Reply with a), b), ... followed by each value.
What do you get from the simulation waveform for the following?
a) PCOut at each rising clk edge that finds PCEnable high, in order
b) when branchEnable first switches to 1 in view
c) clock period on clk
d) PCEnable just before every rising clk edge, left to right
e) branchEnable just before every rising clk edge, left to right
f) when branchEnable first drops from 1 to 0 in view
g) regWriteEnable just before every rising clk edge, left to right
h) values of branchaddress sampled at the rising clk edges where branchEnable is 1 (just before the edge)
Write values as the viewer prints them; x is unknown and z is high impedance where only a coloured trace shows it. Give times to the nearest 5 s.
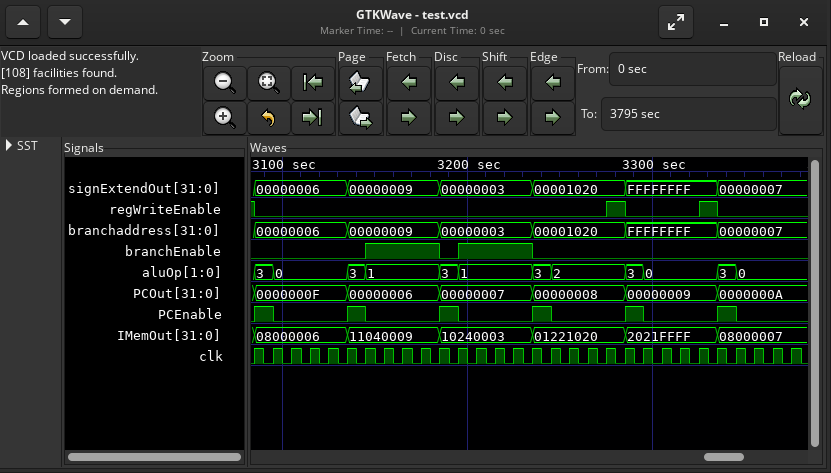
a) 0000000F, 00000006, 00000007, 00000008, 00000009, 0000000A
b) 3145 s
c) 10 s
d) 0 1 0 0 0 0 1 0 0 0 0 1 0 0 0 0 1 0 0 0 0 1 0 0 0 0 1 0 0 0
e) 0 0 0 0 0 0 0 1 1 1 1 0 1 1 1 1 0 0 0 0 0 0 0 0 0 0 0 0 0 0
f) 3185 s
g) 1 0 0 0 0 0 0 0 0 0 0 0 0 0 0 0 0 0 0 0 1 0 0 0 0 1 0 0 0 0
h) 00000009, 00000009, 00000009, 00000009, 00000003, 00000003, 00000003, 00000003
